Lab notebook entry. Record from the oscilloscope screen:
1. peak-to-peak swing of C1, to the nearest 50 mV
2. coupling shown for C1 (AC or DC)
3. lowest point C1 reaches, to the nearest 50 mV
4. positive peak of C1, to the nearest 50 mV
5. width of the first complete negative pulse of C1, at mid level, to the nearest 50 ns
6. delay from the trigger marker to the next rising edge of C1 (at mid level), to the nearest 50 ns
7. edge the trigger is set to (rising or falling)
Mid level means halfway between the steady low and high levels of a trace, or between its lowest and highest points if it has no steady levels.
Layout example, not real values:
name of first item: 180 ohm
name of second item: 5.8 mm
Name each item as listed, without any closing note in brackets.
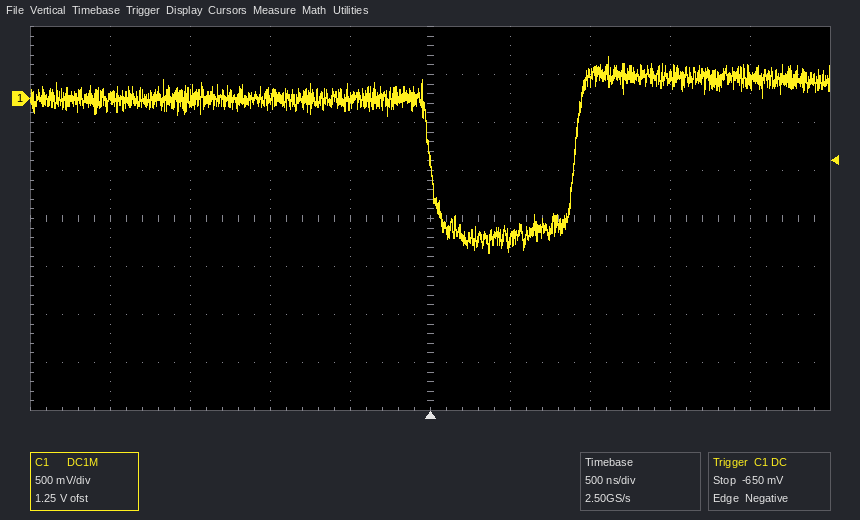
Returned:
peak-to-peak swing of C1, to the nearest 50 mV: 2.05 V
coupling shown for C1: DC
lowest point C1 reaches, to the nearest 50 mV: -1.60 V
positive peak of C1, to the nearest 50 mV: 450 mV
width of the first complete negative pulse of C1, at mid level, to the nearest 50 ns: 900 ns
delay from the trigger marker to the next rising edge of C1 (at mid level), to the nearest 50 ns: 900 ns
edge the trigger is set to: falling
